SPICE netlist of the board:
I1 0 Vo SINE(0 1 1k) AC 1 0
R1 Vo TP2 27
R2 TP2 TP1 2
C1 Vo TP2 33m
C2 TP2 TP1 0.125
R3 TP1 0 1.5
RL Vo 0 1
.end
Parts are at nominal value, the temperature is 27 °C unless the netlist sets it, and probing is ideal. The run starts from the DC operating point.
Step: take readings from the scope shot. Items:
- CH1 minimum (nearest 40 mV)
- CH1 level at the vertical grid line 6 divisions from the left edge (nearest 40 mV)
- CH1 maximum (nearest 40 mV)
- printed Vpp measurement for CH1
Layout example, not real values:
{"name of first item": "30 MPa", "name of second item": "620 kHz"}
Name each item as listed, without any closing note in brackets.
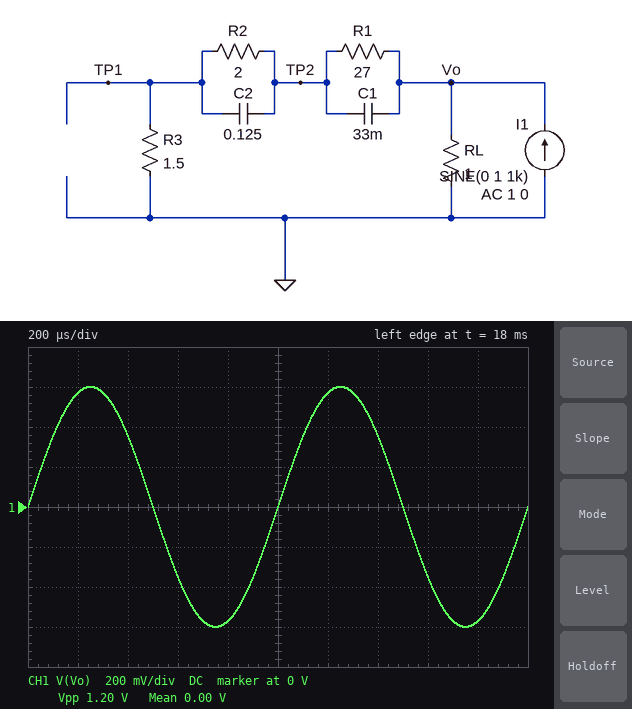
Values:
{"CH1 minimum": "-600 mV", "CH1 level at the vertical grid line 6 divisions from the left edge": "560 mV", "CH1 maximum": "600 mV", "printed Vpp measurement for CH1": "1.20 V"}
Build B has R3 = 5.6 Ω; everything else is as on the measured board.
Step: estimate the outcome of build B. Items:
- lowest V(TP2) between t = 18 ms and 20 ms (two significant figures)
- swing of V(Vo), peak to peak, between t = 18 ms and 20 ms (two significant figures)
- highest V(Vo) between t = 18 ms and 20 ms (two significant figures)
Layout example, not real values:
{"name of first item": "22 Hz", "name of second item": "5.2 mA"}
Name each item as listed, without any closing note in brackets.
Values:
{"lowest V(TP2) between t = 18 ms and 20 ms": "-850 mV", "swing of V(Vo), peak to peak, between t = 18 ms and 20 ms": "1.7 V", "highest V(Vo) between t = 18 ms and 20 ms": "850 mV"}
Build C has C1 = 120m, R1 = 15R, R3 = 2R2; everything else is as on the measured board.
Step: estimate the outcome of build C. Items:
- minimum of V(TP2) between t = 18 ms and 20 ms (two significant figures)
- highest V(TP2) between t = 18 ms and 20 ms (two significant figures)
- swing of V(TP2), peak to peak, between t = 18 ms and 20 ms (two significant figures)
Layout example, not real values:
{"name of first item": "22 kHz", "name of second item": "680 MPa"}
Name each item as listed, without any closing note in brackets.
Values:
{"minimum of V(TP2) between t = 18 ms and 20 ms": "-690 mV", "highest V(TP2) between t = 18 ms and 20 ms": "690 mV", "swing of V(TP2), peak to peak, between t = 18 ms and 20 ms": "1.4 V"}
